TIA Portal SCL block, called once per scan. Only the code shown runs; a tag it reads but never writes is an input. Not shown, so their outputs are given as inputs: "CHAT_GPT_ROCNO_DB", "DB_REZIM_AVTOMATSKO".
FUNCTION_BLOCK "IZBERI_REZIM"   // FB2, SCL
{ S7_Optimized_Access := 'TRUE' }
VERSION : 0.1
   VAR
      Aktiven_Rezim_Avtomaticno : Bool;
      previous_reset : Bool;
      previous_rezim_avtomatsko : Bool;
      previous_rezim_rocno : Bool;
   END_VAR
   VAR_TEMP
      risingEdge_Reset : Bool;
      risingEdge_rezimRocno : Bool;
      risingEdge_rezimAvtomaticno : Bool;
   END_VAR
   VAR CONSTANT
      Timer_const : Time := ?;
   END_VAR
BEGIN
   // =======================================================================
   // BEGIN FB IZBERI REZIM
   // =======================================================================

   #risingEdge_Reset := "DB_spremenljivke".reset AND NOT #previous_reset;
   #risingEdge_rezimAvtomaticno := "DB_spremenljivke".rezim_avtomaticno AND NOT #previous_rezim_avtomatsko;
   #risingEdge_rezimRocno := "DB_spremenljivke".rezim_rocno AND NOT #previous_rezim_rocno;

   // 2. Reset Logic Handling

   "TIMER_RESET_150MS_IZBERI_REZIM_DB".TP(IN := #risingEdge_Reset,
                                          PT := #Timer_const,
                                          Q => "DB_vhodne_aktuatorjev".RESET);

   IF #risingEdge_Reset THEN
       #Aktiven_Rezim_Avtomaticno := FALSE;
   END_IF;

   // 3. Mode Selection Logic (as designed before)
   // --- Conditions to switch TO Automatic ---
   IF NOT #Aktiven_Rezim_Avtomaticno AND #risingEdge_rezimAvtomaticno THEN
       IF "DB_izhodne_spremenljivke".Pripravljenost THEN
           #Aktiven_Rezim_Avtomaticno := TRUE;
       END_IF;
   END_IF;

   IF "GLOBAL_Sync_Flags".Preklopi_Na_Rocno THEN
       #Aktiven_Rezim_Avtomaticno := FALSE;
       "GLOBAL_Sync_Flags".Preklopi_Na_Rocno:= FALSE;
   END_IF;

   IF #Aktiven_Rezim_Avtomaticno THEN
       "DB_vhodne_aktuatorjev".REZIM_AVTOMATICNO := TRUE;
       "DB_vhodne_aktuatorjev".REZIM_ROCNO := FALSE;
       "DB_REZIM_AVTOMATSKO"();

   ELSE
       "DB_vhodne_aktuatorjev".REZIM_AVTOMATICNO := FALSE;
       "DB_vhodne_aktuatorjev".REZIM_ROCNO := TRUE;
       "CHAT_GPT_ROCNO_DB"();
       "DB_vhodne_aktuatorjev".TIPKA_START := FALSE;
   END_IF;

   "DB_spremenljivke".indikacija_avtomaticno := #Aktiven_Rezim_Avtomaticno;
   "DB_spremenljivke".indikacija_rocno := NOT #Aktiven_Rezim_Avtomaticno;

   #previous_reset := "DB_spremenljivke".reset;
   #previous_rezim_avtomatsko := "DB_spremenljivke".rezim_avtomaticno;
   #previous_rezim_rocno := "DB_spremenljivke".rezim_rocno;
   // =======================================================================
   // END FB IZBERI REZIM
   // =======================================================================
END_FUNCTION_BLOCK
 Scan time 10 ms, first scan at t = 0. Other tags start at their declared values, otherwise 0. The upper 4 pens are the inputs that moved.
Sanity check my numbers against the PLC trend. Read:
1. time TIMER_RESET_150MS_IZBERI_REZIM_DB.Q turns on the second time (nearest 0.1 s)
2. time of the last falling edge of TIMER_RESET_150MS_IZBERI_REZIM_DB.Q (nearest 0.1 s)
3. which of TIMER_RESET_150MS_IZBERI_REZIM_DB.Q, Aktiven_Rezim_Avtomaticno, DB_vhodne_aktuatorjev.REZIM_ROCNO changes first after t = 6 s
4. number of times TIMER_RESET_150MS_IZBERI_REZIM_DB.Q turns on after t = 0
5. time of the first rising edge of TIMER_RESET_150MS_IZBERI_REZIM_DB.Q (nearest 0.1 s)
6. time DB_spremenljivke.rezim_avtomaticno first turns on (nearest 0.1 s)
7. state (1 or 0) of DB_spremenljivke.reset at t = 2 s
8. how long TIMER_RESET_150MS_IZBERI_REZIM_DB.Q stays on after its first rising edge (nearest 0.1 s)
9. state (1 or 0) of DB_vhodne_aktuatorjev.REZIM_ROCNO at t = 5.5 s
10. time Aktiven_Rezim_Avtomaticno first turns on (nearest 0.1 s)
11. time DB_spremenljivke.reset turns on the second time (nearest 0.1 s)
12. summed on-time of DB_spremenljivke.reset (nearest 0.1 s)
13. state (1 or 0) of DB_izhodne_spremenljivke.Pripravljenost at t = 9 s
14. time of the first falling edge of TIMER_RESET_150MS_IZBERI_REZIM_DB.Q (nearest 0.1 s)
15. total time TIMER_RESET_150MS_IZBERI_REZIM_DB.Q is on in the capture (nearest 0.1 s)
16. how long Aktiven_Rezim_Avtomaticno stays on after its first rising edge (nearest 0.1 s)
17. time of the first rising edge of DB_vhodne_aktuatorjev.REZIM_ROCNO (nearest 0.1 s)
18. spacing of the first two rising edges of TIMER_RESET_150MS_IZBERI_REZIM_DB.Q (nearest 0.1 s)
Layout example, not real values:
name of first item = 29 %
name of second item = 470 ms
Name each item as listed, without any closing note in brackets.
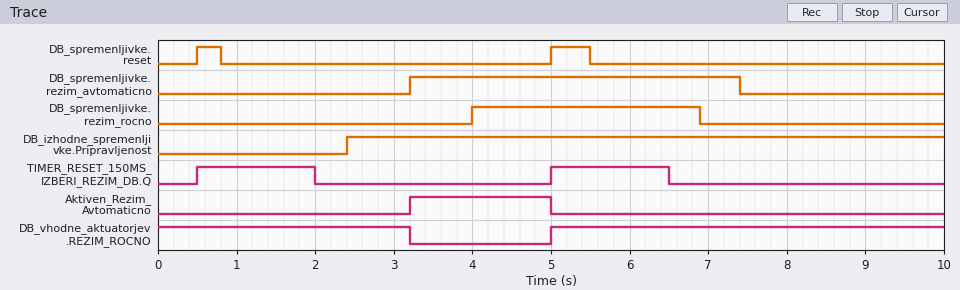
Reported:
time TIMER_RESET_150MS_IZBERI_REZIM_DB.Q turns on the second time = 5.0 s
time of the last falling edge of TIMER_RESET_150MS_IZBERI_REZIM_DB.Q = 6.5 s
which of TIMER_RESET_150MS_IZBERI_REZIM_DB.Q, Aktiven_Rezim_Avtomaticno, DB_vhodne_aktuatorjev.REZIM_ROCNO changes first after t = 6 s = TIMER_RESET_150MS_IZBERI_REZIM_DB.Q
number of times TIMER_RESET_150MS_IZBERI_REZIM_DB.Q turns on after t = 0 = 2
time of the first rising edge of TIMER_RESET_150MS_IZBERI_REZIM_DB.Q = 0.5 s
time DB_spremenljivke.rezim_avtomaticno first turns on = 3.2 s
state (1 or 0) of DB_spremenljivke.reset at t = 2 s = 0
how long TIMER_RESET_150MS_IZBERI_REZIM_DB.Q stays on after its first rising edge = 1.5 s
state (1 or 0) of DB_vhodne_aktuatorjev.REZIM_ROCNO at t = 5.5 s = 1
time Aktiven_Rezim_Avtomaticno first turns on = 3.2 s
time DB_spremenljivke.reset turns on the second time = 5.0 s
summed on-time of DB_spremenljivke.reset = 0.8 s
state (1 or 0) of DB_izhodne_spremenljivke.Pripravljenost at t = 9 s = 1
time of the first falling edge of TIMER_RESET_150MS_IZBERI_REZIM_DB.Q = 2.0 s
total time TIMER_RESET_150MS_IZBERI_REZIM_DB.Q is on in the capture = 3.0 s
how long Aktiven_Rezim_Avtomaticno stays on after its first rising edge = 1.8 s
time of the first rising edge of DB_vhodne_aktuatorjev.REZIM_ROCNO = 5.0 s
spacing of the first two rising edges of TIMER_RESET_150MS_IZBERI_REZIM_DB.Q = 4.5 s
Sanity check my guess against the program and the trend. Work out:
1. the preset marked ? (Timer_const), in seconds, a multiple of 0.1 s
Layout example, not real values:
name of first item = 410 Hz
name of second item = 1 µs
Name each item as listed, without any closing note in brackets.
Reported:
the preset marked ? (Timer_const), in seconds, a multiple of 0.1 s = 1.5 s
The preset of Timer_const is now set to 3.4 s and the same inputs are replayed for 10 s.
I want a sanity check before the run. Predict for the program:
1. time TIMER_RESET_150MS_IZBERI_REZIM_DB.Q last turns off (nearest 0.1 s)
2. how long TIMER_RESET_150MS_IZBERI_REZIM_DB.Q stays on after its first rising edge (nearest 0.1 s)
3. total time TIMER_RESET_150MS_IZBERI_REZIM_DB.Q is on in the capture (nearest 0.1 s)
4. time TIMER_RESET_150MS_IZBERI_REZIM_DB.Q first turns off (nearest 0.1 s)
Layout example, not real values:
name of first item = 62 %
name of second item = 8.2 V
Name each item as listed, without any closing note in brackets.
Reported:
time TIMER_RESET_150MS_IZBERI_REZIM_DB.Q last turns off = 8.4 s
how long TIMER_RESET_150MS_IZBERI_REZIM_DB.Q stays on after its first rising edge = 3.4 s
total time TIMER_RESET_150MS_IZBERI_REZIM_DB.Q is on in the capture = 6.8 s
time TIMER_RESET_150MS_IZBERI_REZIM_DB.Q first turns off = 3.9 s
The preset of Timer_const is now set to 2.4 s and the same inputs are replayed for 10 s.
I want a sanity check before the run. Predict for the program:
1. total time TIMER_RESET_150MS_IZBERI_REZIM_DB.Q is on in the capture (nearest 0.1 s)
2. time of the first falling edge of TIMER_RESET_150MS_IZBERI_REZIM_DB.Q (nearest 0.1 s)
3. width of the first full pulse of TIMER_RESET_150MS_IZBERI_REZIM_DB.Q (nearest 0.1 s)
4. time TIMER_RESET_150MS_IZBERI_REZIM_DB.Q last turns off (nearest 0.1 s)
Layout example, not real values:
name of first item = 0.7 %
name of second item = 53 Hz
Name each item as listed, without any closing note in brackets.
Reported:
total time TIMER_RESET_150MS_IZBERI_REZIM_DB.Q is on in the capture = 4.8 s
time of the first falling edge of TIMER_RESET_150MS_IZBERI_REZIM_DB.Q = 2.9 s
width of the first full pulse of TIMER_RESET_150MS_IZBERI_REZIM_DB.Q = 2.4 s
time TIMER_RESET_150MS_IZBERI_REZIM_DB.Q last turns off = 7.4 s
